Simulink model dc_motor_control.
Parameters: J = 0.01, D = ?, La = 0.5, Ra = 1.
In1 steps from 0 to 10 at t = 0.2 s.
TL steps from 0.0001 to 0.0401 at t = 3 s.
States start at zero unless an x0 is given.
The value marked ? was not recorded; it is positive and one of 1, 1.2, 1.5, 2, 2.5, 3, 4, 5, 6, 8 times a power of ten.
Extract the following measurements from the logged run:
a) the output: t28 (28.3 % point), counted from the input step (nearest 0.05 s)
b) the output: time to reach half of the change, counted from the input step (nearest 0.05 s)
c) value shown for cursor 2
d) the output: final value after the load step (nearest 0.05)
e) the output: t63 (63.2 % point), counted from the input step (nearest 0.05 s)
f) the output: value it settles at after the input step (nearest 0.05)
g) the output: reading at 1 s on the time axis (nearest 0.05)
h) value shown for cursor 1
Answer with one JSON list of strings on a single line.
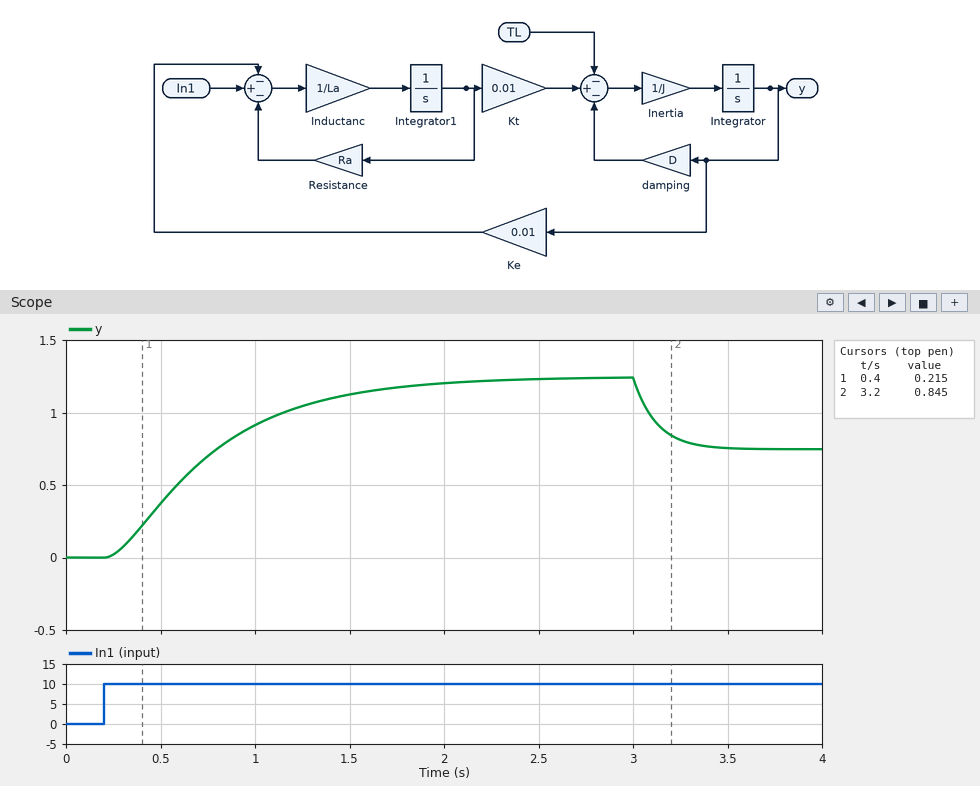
["0.30 s", "0.50 s", "0.845", "0.75", "0.65 s", "1.25", "0.90", "0.215"]
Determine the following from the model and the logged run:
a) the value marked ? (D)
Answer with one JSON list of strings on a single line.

["0.08"]
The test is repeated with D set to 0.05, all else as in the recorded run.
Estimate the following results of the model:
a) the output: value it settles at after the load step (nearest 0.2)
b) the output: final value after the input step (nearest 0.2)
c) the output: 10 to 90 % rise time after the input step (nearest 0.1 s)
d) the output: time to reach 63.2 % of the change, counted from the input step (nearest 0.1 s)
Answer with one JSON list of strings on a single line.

["1.2", "2.0", "1.2 s", "0.7 s"]
